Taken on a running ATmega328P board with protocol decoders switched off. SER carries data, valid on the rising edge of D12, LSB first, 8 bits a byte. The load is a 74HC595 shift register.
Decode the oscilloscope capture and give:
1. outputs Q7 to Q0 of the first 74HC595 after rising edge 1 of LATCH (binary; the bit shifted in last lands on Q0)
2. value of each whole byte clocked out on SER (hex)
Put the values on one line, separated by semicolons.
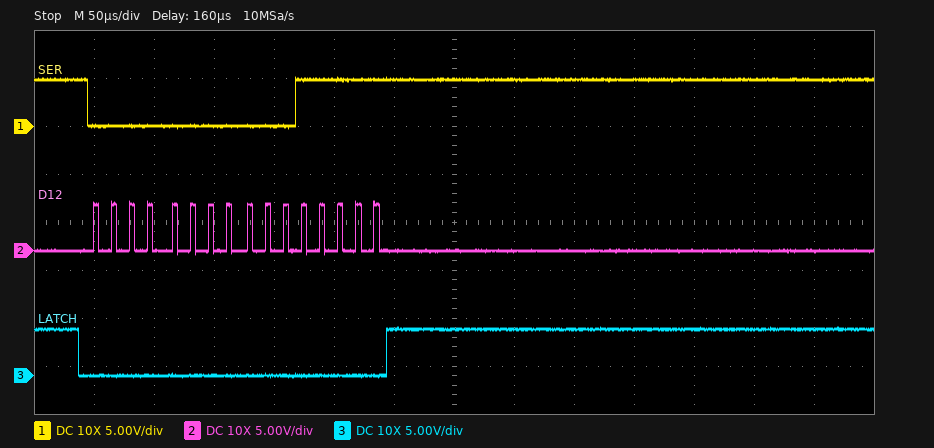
00011111; 00 F8
